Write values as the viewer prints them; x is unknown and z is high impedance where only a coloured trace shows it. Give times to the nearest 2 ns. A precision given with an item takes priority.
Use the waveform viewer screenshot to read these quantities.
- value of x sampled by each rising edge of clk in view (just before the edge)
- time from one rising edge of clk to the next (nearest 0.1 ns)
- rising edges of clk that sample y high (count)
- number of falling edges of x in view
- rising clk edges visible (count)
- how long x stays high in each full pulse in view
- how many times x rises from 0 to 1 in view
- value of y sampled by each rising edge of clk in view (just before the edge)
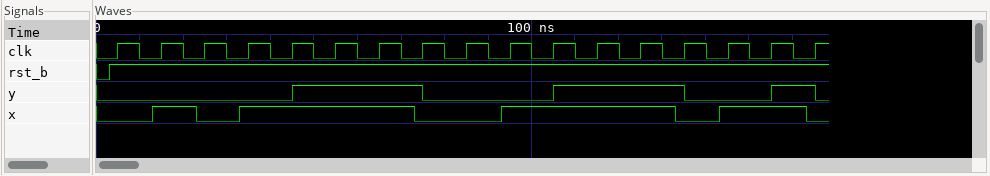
0 1 0 1 1 1 1 0 0 1 1 1 1 0 1 1 0
10 ns
7
4
17
10 ns, 40 ns, 40 ns, 20 ns
4
0 0 0 0 0 1 1 1 0 0 0 1 1 1 0 0 1
